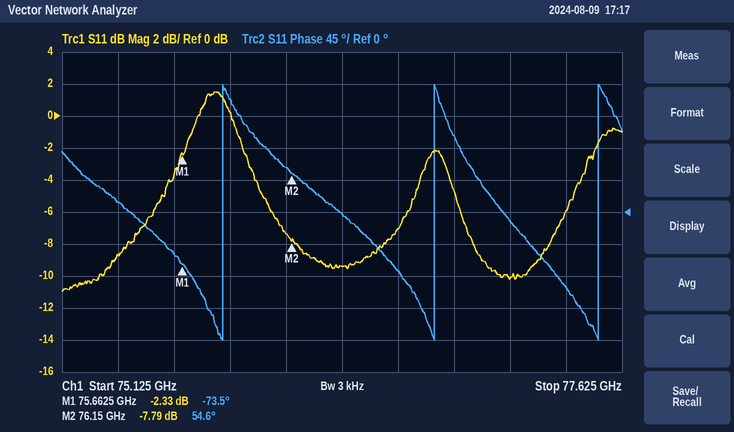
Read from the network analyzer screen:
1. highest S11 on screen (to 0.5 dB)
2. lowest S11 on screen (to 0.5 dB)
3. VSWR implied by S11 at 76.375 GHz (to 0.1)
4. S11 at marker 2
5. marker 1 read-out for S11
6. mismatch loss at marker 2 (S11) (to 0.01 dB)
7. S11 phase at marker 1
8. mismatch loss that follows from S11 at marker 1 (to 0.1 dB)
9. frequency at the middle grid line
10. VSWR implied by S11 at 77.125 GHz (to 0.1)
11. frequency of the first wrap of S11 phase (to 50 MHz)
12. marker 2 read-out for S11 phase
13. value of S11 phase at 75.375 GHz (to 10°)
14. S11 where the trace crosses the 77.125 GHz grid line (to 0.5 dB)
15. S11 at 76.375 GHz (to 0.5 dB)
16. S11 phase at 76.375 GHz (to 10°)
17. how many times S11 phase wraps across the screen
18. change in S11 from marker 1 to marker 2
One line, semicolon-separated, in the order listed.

1.5 dB; -11.0 dB; 2.0; -7.79 dB; -2.33 dB; 0.79 dB; -73.5°; 3.8 dB; 76.375 GHz; 1.9; 75.85 GHz; 54.6°; 10°; -10.0 dB; -9.5 dB; 0°; 3; -5.46 dB
